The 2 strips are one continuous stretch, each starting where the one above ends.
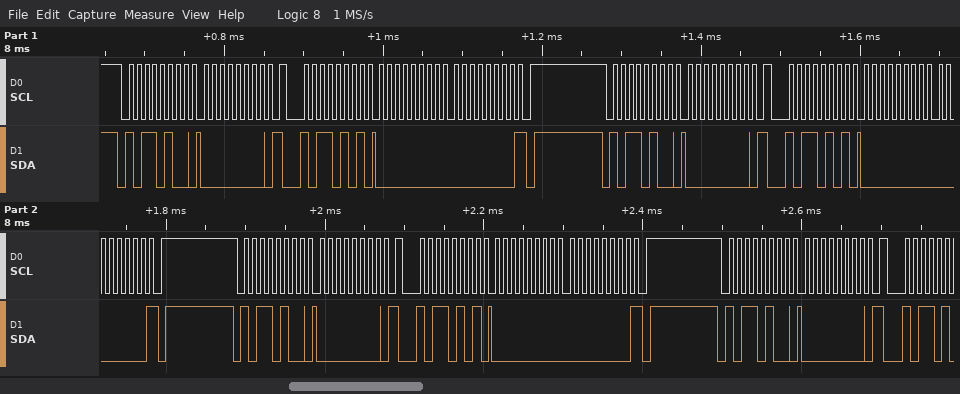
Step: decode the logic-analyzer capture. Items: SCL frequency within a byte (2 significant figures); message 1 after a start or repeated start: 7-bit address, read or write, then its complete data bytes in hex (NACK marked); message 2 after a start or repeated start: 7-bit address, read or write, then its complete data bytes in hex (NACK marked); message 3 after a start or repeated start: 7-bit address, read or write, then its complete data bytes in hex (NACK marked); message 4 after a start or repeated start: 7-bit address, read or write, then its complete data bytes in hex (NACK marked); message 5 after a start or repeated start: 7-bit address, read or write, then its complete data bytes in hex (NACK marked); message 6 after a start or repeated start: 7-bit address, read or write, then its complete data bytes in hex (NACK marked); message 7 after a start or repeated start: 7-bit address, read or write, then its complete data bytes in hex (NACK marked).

100 kHz
0x5A write: 00
0x5A read: 00 00 NACK
0x5A write: 00
0x5A read: 00 00 NACK
0x5A write: 00
0x5A read: 00 00 NACK
0x5A write: 00
